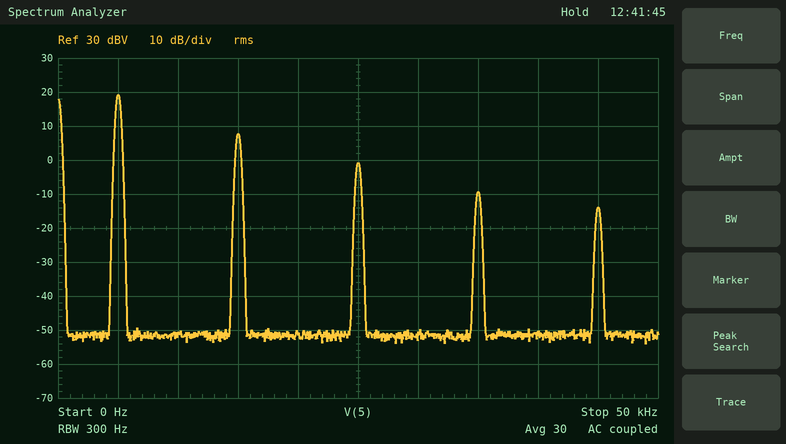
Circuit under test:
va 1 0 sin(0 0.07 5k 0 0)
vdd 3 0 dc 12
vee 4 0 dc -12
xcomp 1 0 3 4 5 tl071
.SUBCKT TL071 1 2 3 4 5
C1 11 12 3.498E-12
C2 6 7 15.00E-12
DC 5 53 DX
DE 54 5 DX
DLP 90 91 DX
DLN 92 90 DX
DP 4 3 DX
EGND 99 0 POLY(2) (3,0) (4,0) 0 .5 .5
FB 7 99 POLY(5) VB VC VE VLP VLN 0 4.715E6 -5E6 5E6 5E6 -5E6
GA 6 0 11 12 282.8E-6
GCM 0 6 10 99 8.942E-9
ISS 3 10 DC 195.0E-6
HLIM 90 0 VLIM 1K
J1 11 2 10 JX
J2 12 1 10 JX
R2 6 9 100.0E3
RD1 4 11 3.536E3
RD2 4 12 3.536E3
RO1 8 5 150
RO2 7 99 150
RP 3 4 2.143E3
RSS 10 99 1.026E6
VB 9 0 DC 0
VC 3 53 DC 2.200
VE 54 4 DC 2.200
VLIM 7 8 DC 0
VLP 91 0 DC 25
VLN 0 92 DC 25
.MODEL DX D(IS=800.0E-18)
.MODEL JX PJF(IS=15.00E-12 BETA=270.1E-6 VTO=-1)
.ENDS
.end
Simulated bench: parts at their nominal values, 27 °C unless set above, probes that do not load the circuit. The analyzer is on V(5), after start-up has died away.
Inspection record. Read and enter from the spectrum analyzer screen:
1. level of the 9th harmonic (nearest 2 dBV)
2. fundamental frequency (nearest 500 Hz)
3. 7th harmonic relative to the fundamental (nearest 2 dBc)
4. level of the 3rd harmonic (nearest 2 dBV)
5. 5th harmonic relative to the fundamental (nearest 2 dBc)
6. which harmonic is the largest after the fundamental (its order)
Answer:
-14 dBV
5.0 kHz
-28 dBc
8 dBV
-20 dBc
3
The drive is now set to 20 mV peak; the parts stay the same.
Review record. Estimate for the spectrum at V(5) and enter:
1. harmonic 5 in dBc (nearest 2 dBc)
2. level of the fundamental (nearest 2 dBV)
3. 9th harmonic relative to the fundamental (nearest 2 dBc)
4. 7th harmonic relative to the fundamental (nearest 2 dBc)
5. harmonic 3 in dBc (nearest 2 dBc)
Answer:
-30 dBc
18 dBV
-42 dBc
-38 dBc
-20 dBc
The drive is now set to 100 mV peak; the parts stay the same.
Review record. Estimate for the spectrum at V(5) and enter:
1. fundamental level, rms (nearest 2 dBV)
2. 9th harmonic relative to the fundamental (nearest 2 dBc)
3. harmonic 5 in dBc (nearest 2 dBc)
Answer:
20 dBV
-32 dBc
-18 dBc
